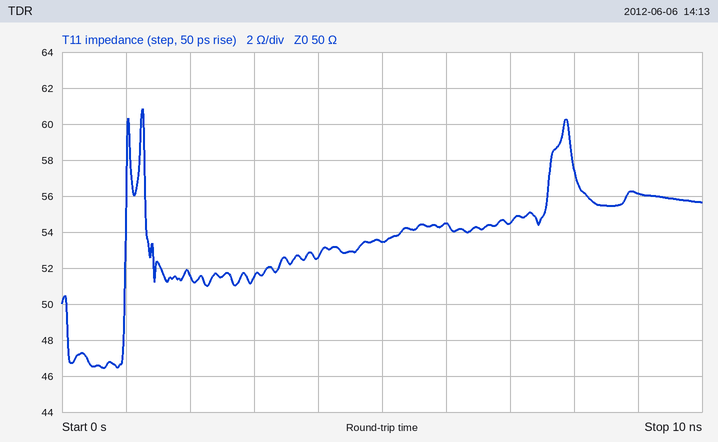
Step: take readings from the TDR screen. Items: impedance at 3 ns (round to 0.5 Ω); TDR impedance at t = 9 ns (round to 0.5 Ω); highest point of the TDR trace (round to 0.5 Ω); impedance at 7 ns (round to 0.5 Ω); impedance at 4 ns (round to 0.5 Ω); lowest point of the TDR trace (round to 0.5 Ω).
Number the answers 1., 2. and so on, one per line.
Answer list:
1. 51.5 Ω
2. 56.0 Ω
3. 61.0 Ω
4. 54.5 Ω
5. 52.5 Ω
6. 46.5 Ω
